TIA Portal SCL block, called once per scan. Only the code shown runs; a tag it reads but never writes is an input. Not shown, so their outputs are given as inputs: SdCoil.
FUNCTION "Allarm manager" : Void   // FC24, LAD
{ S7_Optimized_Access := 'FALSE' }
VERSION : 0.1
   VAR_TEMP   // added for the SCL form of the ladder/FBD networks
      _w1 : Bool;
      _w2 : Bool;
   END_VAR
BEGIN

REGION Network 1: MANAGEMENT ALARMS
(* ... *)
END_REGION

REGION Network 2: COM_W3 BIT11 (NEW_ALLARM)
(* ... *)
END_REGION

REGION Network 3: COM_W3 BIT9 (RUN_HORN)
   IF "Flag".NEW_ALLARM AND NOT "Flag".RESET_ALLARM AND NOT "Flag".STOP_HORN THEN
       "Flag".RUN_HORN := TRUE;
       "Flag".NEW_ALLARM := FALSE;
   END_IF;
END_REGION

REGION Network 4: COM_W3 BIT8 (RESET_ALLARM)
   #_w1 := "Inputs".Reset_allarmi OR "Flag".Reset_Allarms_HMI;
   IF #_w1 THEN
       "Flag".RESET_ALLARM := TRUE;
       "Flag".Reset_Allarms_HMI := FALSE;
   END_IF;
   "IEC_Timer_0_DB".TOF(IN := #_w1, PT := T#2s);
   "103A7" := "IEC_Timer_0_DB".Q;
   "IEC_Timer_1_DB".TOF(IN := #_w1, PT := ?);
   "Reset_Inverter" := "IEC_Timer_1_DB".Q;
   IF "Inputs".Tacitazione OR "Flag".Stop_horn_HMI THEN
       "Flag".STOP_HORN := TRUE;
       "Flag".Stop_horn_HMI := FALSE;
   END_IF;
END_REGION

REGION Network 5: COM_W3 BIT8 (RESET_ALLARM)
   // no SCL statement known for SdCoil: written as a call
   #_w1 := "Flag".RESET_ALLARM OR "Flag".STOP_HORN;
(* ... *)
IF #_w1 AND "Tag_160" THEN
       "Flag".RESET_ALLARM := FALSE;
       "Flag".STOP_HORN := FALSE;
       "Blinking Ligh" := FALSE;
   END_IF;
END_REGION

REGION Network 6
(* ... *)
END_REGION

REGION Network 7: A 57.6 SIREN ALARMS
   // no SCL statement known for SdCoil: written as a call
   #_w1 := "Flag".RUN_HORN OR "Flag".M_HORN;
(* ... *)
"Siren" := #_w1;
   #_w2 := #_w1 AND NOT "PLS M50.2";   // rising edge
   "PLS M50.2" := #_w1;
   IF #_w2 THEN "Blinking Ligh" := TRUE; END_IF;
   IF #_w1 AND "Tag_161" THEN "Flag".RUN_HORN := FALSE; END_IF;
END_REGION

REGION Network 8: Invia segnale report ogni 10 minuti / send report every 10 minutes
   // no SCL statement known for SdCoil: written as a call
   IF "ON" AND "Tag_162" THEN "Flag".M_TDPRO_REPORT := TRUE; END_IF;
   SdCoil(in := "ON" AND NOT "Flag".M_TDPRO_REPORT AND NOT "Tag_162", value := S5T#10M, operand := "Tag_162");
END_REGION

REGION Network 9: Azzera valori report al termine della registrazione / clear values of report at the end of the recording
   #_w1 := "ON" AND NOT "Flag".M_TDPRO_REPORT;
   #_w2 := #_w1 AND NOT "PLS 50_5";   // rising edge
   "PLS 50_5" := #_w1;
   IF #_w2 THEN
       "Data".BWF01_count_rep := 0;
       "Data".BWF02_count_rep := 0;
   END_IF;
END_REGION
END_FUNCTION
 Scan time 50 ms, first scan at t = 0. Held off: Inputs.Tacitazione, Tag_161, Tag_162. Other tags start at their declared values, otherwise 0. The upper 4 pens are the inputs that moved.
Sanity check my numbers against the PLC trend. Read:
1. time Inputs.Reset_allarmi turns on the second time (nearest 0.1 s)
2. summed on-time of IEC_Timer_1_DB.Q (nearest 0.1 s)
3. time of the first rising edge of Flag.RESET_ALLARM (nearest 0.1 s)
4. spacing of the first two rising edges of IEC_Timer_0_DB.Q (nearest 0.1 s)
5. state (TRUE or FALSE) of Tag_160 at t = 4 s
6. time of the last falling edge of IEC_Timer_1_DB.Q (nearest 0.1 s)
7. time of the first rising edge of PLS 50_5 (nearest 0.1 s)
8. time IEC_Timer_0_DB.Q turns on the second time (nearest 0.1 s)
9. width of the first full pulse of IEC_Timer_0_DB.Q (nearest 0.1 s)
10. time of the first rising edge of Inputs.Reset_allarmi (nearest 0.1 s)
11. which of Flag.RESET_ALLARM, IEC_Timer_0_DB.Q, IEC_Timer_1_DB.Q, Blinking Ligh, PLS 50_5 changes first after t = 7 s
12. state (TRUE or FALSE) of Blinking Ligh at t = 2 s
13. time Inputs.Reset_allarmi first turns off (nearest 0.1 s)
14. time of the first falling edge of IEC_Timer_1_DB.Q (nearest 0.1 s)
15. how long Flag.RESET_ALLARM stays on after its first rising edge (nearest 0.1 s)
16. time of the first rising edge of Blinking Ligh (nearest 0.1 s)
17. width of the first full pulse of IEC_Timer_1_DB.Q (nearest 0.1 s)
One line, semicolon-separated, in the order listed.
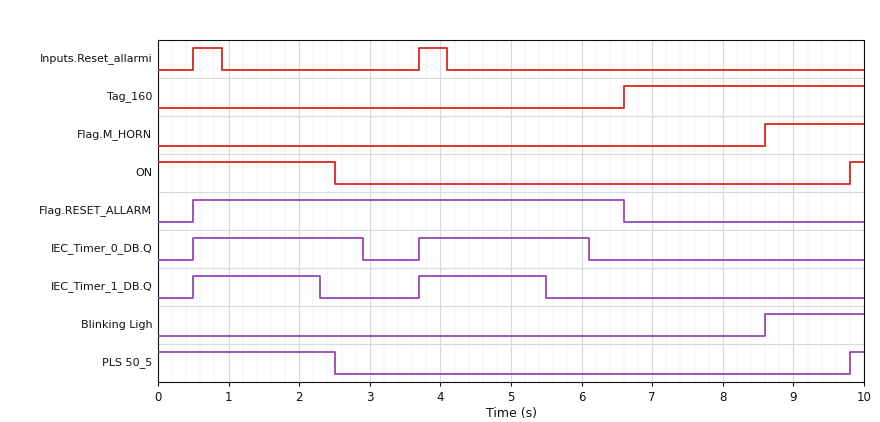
3.7 s; 3.6 s; 0.5 s; 3.2 s; FALSE; 5.5 s; 9.8 s; 3.7 s; 2.4 s; 0.5 s; Blinking Ligh; FALSE; 0.9 s; 2.3 s; 6.1 s; 8.6 s; 1.8 s
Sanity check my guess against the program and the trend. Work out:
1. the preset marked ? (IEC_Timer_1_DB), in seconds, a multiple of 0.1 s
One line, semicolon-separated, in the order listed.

1.4 s
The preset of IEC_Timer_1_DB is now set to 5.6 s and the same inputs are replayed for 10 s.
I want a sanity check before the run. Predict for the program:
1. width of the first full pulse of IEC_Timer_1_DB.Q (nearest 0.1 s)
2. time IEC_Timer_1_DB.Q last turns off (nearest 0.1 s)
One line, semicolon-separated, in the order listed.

9.2 s; 9.7 s
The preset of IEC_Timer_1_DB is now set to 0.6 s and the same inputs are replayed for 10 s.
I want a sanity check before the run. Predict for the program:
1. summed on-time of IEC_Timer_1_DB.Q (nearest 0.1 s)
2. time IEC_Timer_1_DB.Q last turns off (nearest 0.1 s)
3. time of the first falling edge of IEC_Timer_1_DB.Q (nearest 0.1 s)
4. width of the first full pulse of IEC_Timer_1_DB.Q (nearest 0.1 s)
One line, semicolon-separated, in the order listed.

2.0 s; 4.7 s; 1.5 s; 1.0 s
